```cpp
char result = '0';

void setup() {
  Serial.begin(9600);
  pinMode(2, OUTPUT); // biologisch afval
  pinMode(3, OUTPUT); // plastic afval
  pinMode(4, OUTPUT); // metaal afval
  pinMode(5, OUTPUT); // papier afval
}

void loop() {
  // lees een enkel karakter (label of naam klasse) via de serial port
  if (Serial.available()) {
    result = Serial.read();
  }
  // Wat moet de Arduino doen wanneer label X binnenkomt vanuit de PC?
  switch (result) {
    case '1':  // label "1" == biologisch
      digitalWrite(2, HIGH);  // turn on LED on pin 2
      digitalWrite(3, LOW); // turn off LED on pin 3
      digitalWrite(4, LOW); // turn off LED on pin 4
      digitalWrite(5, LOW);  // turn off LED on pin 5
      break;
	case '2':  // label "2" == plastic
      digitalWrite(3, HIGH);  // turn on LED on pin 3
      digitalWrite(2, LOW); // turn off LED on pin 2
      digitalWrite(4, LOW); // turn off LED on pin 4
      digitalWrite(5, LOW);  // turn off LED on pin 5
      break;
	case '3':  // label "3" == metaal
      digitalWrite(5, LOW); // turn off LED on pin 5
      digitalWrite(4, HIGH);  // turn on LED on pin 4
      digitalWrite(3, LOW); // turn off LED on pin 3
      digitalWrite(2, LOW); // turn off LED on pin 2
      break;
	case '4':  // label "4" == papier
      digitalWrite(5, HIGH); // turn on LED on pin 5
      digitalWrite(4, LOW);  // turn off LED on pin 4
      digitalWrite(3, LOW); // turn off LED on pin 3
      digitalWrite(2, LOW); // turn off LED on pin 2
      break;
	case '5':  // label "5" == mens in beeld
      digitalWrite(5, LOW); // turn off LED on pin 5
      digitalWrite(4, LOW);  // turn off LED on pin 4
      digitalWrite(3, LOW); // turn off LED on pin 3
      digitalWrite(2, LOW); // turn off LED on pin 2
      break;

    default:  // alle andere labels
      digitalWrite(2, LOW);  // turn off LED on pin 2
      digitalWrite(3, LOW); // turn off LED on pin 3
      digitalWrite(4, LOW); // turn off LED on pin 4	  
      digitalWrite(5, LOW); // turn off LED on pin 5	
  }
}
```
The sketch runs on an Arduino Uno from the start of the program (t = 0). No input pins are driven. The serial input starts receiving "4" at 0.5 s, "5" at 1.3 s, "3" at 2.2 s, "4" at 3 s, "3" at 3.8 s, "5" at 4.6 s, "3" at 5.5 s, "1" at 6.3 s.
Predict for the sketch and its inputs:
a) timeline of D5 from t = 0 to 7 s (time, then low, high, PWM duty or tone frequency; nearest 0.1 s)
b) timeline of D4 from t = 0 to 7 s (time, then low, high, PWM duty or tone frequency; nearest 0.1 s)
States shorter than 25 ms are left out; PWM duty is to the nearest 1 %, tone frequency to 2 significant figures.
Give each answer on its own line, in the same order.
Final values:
0 s low; 0.5 s high; 1.3 s low; 3 s high; 3.8 s low
0 s low; 2.2 s high; 3 s low; 3.8 s high; 4.6 s low; 5.5 s high; 6.3 s low
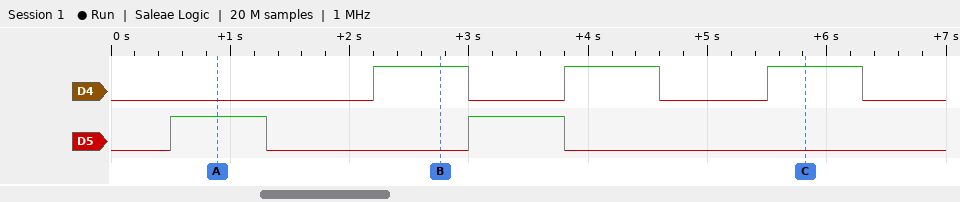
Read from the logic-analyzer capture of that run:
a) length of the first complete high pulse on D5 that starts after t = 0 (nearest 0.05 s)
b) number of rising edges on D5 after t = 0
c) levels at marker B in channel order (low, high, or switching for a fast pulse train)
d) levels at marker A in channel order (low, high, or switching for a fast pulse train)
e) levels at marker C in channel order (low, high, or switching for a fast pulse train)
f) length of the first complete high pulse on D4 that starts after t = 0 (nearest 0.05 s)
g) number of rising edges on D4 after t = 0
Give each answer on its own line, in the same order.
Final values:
0.80 s
2
D4 high, D5 low
D4 low, D5 high
D4 high, D5 low
0.80 s
3
